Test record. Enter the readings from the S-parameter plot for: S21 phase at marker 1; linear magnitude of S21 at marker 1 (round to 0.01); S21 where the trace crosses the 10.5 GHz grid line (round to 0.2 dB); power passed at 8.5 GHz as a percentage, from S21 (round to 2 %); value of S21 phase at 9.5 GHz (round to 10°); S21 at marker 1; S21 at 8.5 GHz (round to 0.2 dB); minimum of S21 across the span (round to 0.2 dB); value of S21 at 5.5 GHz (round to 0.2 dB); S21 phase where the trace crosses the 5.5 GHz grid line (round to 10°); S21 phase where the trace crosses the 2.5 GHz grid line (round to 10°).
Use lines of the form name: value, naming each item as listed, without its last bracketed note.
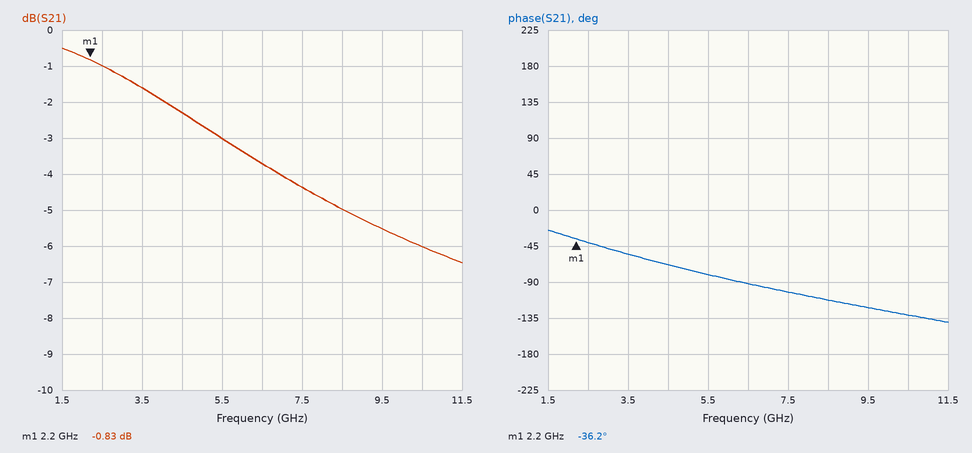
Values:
S21 phase at marker 1: -36.2°
linear magnitude of S21 at marker 1: 0.91
S21 where the trace crosses the 10.5 GHz grid line: -6.0 dB
power passed at 8.5 GHz as a percentage, from S21: 32 %
value of S21 phase at 9.5 GHz: -120°
S21 at marker 1: -0.83 dB
S21 at 8.5 GHz: -5.0 dB
minimum of S21 across the span: -6.4 dB
value of S21 at 5.5 GHz: -3.0 dB
S21 phase where the trace crosses the 5.5 GHz grid line: -80°
S21 phase where the trace crosses the 2.5 GHz grid line: -40°
